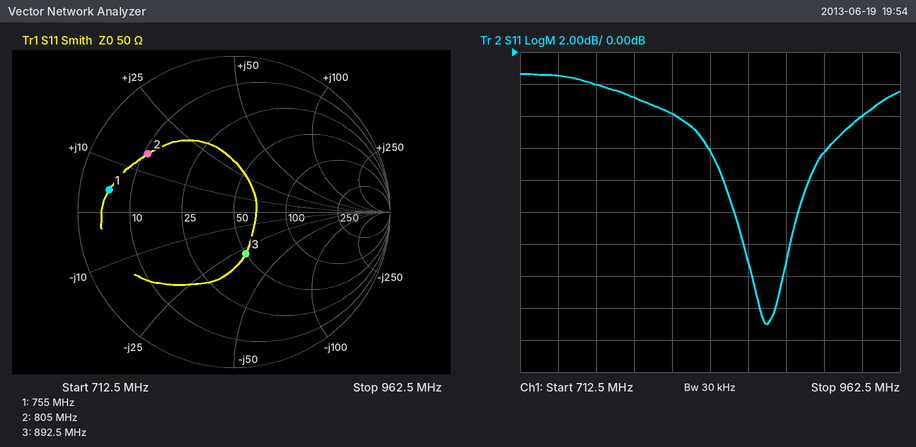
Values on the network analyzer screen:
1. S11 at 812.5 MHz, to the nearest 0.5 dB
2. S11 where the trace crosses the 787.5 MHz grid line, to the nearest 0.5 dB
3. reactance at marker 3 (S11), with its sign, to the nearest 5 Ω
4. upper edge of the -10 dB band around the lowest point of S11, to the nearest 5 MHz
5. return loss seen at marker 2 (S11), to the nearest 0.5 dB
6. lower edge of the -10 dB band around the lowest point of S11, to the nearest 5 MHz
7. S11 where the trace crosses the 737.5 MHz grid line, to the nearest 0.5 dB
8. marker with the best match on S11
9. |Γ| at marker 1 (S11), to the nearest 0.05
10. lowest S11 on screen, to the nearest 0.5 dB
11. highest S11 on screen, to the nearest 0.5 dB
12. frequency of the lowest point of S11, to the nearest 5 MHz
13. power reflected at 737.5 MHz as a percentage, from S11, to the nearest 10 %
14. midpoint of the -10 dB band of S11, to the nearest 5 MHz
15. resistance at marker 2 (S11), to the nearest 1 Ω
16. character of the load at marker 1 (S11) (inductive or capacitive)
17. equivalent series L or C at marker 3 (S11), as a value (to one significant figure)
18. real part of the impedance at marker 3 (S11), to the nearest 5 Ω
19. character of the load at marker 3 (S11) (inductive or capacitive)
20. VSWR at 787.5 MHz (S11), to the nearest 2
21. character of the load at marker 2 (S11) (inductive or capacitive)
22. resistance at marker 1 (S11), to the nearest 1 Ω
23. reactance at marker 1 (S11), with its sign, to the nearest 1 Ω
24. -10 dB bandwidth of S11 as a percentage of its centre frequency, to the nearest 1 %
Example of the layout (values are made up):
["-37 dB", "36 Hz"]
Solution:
["-4.0 dB", "-3.0 dB", "-30 Ω", "895 MHz", "3.5 dB", "855 MHz", "-1.5 dB", "marker 3", "0.80", "-17.0 dB", "-1.5 dB", "875 MHz", "70 %", "875 MHz", "11 Ω", "inductive", "6 pF", "50 Ω", "capacitive", "6", "inductive", "5 Ω", "+4 Ω", "5 %"]
